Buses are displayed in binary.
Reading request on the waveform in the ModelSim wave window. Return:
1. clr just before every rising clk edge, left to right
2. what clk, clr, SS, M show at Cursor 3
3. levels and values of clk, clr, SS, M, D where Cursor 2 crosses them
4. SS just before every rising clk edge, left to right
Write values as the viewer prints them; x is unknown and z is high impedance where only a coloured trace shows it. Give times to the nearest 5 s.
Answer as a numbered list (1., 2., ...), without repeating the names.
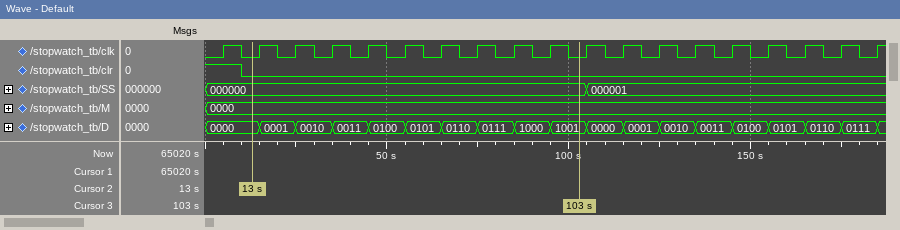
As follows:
1. 1 0 0 0 0 0 0 0 0 0 0 0 0 0 0 0 0 0 0
2. clk=0, clr=0, SS=000000, M=0000
3. clk=0, clr=0, SS=000000, M=0000, D=0000
4. 000000, 000000, 000000, 000000, 000000, 000000, 000000, 000000, 000000, 000000, 000000, 000001, 000001, 000001, 000001, 000001, 000001, 000001, 000001
